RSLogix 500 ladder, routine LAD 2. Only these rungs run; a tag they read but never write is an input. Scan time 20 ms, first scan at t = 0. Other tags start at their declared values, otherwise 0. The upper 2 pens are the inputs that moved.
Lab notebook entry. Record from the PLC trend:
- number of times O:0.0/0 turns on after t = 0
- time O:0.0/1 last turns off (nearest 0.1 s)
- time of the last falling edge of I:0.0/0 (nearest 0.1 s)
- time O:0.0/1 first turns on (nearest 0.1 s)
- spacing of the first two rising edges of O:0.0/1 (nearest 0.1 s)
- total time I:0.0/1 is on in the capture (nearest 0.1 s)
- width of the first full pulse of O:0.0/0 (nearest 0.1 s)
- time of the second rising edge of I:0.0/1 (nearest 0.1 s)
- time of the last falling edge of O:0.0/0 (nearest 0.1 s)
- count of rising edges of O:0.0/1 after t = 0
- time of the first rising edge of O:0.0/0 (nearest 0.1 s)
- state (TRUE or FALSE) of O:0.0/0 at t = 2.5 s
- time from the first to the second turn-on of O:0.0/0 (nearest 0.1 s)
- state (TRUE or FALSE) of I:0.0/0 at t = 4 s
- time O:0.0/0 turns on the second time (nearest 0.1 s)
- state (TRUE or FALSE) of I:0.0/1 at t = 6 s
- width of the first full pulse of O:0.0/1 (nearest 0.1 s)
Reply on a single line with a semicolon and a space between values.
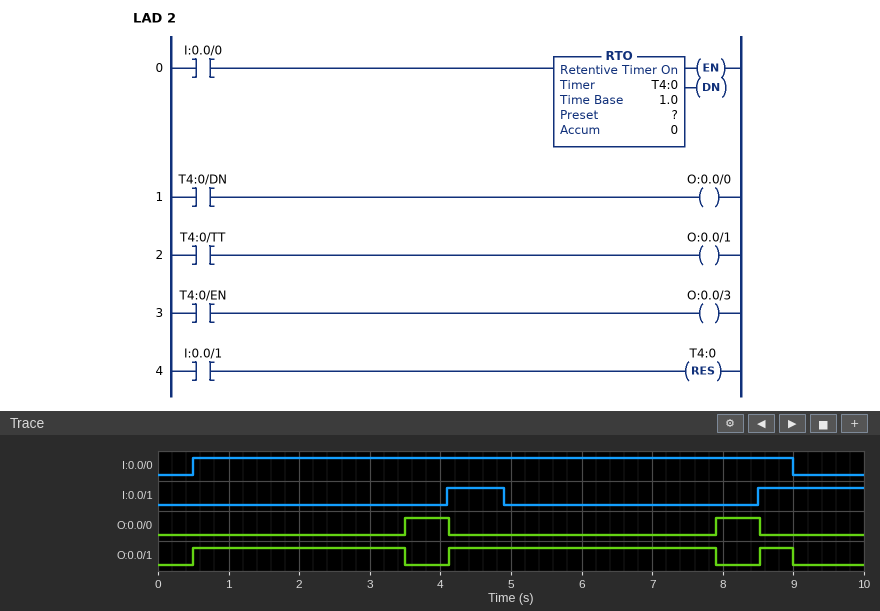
2; 9.0 s; 9.0 s; 0.5 s; 3.6 s; 2.3 s; 0.6 s; 8.5 s; 8.5 s; 3; 3.5 s; FALSE; 4.4 s; TRUE; 7.9 s; FALSE; 3.0 s
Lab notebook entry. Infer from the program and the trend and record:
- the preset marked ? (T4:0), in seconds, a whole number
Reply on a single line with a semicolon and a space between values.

3 s
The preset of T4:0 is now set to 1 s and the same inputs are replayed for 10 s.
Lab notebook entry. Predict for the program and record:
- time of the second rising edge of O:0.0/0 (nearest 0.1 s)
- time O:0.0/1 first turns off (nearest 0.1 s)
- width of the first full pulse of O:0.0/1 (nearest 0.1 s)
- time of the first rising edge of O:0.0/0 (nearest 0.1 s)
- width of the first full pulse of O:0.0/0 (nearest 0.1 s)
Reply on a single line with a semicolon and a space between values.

5.9 s; 1.5 s; 1.0 s; 1.5 s; 2.6 s
